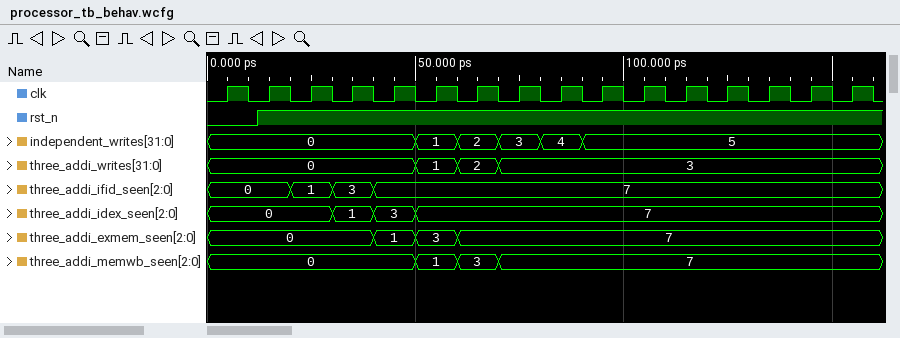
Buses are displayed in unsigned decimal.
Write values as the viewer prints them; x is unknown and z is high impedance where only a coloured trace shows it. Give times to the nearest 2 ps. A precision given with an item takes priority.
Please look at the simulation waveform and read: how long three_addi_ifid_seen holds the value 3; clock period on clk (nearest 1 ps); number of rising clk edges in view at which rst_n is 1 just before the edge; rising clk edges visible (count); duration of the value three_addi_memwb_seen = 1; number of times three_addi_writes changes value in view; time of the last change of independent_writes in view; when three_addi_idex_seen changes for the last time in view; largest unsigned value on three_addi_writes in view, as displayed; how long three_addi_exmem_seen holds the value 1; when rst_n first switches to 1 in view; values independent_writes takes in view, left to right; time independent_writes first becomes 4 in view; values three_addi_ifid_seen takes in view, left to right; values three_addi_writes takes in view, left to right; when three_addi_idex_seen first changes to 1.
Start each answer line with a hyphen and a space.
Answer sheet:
- 10 ps
- 10 ps
- 15
- 16
- 10 ps
- 3
- 90 ps
- 50 ps
- 3
- 10 ps
- 12 ps
- 0, 1, 2, 3, 4, 5
- 80 ps
- 0, 1, 3, 7
- 0, 1, 2, 3
- 30 ps
